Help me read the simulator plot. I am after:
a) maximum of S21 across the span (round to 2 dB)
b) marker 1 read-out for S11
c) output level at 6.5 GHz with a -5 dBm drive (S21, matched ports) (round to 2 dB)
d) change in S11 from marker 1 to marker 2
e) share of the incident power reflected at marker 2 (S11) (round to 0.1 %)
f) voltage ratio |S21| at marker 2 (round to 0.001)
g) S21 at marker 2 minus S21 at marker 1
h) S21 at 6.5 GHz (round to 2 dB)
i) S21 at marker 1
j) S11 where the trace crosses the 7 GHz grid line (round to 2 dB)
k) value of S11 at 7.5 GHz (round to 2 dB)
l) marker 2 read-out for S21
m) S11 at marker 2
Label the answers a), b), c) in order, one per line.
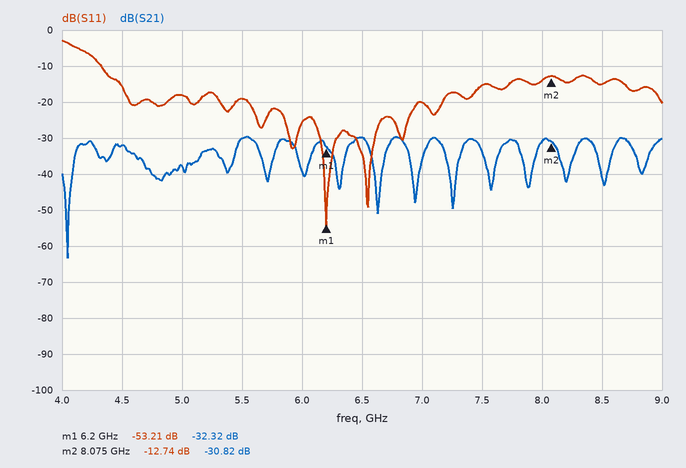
a) -30 dB
b) -53.21 dB
c) -34 dBm
d) 40.47 dB
e) 5.3 %
f) 0.029
g) 1.50 dB
h) -30 dB
i) -32.32 dB
j) -20 dB
k) -16 dB
l) -30.82 dB
m) -12.74 dB
